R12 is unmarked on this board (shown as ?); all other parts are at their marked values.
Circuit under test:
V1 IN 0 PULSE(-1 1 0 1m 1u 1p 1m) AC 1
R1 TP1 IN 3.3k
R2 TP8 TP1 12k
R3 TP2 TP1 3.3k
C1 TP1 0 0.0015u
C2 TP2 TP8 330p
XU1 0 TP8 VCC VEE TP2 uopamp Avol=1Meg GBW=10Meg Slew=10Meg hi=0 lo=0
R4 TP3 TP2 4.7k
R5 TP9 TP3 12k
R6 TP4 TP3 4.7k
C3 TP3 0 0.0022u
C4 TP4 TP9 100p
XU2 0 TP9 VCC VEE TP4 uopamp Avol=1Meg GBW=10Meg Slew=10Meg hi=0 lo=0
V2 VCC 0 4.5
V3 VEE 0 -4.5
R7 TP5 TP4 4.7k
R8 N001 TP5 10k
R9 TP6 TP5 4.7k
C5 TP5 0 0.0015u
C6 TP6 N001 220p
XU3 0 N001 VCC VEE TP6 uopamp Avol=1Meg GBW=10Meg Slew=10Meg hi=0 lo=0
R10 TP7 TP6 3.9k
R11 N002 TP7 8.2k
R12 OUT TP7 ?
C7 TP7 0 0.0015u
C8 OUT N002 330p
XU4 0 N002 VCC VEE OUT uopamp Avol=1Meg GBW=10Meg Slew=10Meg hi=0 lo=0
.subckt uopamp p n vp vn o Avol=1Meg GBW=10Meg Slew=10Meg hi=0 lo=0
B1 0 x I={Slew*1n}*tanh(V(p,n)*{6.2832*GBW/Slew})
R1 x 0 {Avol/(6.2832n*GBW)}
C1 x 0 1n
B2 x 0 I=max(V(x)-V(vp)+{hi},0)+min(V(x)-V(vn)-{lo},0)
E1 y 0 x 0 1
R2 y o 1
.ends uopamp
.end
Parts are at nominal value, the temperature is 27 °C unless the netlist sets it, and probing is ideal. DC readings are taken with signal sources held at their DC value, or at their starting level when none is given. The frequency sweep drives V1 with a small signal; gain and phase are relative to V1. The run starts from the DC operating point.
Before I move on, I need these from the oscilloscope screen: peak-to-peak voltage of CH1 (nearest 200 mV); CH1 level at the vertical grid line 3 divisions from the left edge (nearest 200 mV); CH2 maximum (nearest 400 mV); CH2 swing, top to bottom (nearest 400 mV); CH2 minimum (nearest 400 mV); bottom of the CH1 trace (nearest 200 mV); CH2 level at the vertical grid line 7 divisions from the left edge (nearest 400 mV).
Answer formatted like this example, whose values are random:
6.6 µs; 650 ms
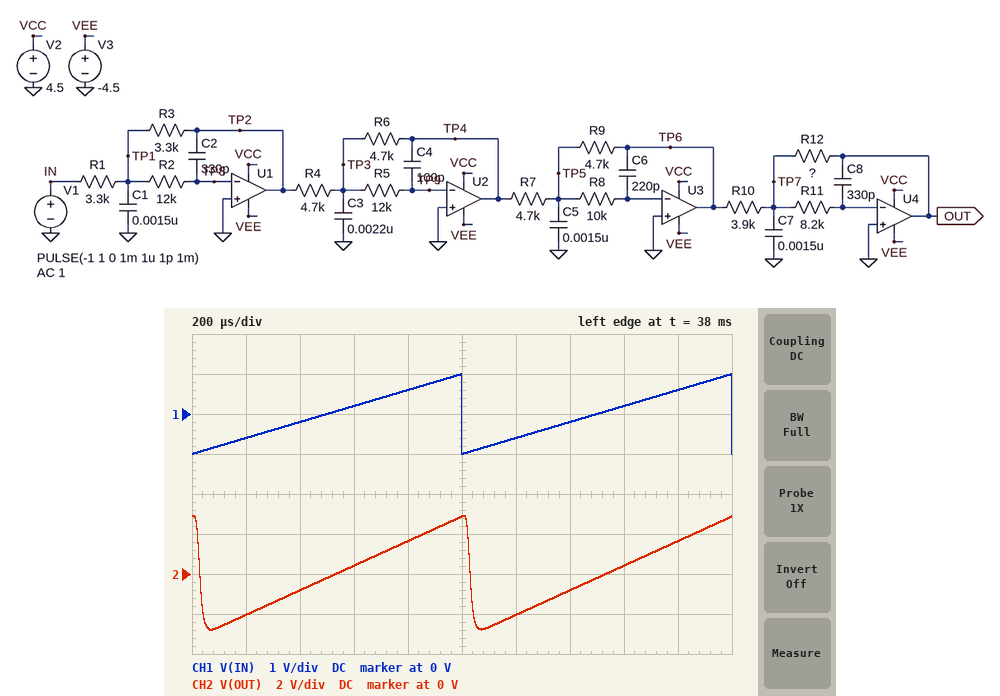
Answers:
2.0 V; 200 mV; 2.8 V; 5.6 V; -2.8 V; -1.0 V; -800 mV
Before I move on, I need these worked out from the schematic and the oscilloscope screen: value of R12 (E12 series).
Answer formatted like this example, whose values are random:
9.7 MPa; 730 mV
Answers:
12 kΩ
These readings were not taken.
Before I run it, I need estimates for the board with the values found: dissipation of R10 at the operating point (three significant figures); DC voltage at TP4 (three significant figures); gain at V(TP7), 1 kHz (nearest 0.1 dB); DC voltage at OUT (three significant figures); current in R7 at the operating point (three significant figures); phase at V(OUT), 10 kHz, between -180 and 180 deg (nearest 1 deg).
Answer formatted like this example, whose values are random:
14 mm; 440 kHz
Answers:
256 µW; -1.00 V; -25.6 dB; -3.08 V; 213 µA; -112 deg
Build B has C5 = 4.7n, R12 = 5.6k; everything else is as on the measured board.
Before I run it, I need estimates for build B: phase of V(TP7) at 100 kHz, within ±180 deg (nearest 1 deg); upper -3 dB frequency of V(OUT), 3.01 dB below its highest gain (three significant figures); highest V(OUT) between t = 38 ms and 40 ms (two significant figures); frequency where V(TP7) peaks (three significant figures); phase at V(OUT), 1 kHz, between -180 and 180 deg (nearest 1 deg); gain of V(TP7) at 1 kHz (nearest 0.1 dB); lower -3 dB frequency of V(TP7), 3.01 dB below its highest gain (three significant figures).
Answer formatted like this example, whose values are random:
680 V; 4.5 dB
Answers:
17 deg; 23.6 kHz; 1.4 V; 20.3 kHz; -9 deg; -32.2 dB; 12.9 kHz
